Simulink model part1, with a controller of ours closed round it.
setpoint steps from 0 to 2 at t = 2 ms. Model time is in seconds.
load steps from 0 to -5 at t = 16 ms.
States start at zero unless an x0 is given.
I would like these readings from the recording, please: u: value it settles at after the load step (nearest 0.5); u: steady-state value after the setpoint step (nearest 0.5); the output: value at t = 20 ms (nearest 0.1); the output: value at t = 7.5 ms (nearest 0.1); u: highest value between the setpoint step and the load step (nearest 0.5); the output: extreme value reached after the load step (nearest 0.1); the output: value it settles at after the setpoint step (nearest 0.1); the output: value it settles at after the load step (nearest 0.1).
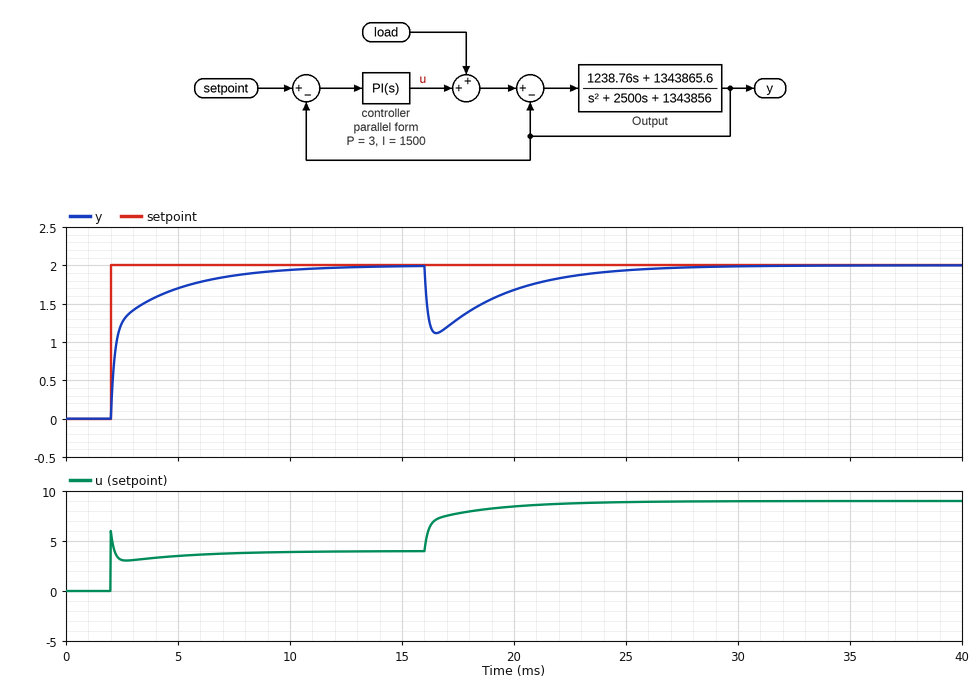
9.0
4.0
1.7
1.9
6.0
1.1
2.0
2.0
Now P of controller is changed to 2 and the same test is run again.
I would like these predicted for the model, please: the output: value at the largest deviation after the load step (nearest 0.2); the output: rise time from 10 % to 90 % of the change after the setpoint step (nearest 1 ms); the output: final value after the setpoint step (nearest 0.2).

1.0
4 ms
2.0
